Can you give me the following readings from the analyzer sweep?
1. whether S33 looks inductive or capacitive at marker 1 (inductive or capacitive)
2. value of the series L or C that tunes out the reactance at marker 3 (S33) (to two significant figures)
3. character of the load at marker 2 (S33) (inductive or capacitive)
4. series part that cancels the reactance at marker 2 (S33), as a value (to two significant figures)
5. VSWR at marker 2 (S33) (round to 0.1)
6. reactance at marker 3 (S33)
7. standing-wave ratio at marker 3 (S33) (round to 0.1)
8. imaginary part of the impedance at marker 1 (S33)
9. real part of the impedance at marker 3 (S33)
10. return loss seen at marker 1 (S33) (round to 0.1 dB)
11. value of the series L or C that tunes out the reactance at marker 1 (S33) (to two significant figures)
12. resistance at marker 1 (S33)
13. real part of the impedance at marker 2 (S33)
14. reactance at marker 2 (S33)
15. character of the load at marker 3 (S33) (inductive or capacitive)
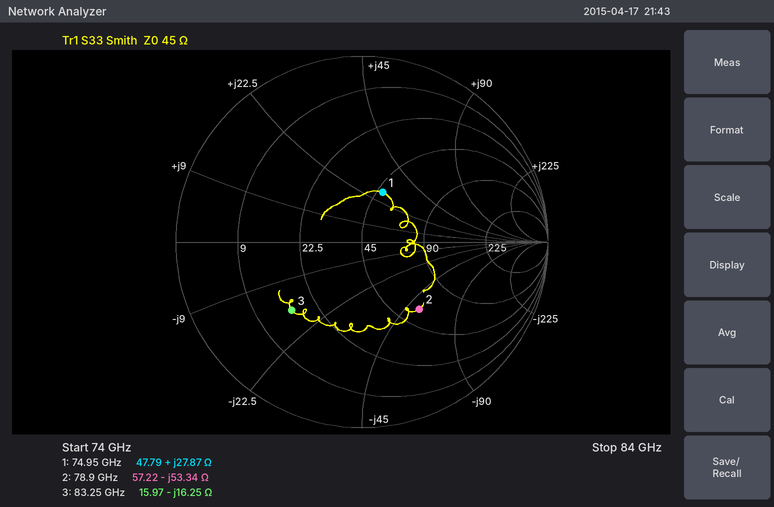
inductive
31 pH
capacitive
110 pH
2.8
-16.25 Ω
3.2
+27.87 Ω
15.97 Ω
10.8 dB
76 fF
47.79 Ω
57.22 Ω
-53.34 Ω
capacitive
